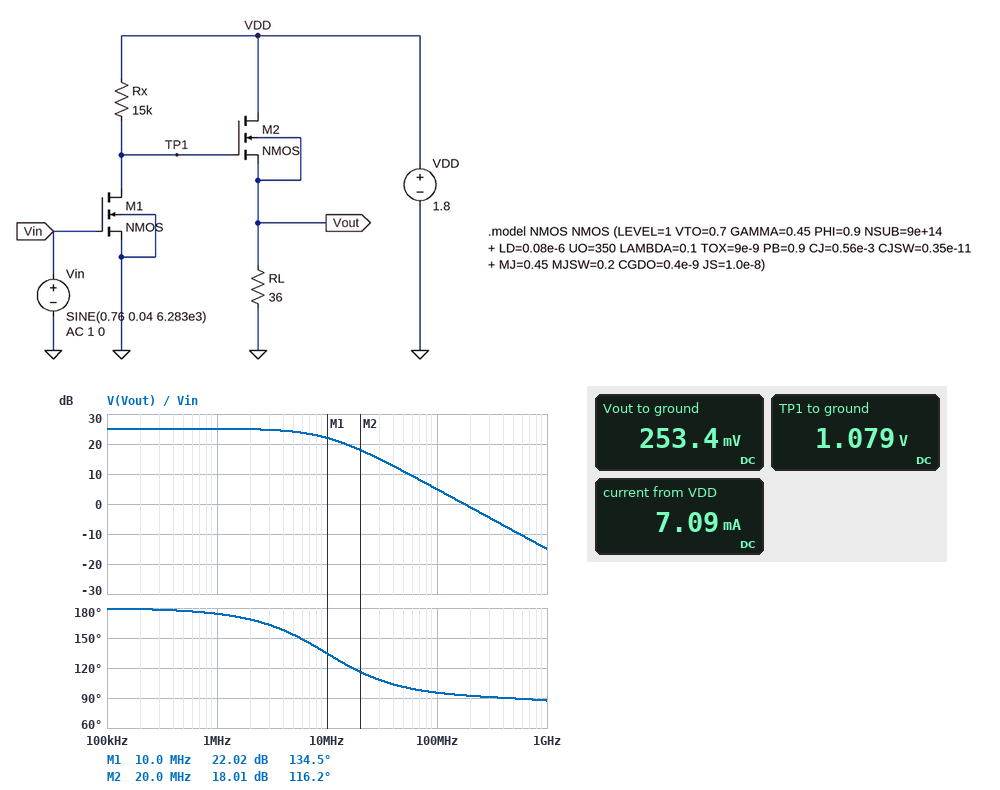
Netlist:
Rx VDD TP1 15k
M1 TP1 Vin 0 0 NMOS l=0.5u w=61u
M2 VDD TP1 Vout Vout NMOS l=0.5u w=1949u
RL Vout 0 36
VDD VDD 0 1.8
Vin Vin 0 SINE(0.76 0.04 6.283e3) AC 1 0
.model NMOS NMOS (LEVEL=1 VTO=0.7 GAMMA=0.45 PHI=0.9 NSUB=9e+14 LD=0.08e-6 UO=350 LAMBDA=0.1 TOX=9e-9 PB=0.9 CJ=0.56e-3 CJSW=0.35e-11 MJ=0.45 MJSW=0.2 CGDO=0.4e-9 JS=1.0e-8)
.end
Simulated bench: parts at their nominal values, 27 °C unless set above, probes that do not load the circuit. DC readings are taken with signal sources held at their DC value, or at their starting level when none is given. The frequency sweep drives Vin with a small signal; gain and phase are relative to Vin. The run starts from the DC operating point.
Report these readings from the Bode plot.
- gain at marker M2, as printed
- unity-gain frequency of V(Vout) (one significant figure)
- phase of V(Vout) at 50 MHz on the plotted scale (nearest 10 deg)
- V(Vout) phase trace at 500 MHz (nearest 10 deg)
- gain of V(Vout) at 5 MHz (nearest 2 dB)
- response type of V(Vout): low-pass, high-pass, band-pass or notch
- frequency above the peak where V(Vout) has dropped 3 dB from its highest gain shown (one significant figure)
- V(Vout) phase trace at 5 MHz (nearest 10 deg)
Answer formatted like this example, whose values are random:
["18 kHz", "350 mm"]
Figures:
["18.01 dB", "200 MHz", "100 deg", "90 deg", "24 dB", "low-pass", "10 MHz", "150 deg"]
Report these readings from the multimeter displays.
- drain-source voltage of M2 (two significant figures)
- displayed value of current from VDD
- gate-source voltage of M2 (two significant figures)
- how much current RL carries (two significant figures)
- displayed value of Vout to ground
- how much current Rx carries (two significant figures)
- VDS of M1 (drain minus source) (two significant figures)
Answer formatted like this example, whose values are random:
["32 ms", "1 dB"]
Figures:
["1.5 V", "7.09 mA", "830 mV", "7.0 mA", "253.4 mV", "48 µA", "1.1 V"]
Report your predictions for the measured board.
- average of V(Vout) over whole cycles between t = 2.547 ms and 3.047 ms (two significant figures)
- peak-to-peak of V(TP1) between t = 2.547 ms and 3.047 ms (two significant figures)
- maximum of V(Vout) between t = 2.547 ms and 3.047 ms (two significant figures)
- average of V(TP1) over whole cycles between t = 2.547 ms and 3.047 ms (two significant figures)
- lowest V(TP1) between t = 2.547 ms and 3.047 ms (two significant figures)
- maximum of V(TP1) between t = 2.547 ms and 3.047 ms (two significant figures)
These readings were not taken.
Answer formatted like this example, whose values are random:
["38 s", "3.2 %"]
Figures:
["330 mV", "1.6 V", "790 mV", "970 mV", "77 mV", "1.7 V"]
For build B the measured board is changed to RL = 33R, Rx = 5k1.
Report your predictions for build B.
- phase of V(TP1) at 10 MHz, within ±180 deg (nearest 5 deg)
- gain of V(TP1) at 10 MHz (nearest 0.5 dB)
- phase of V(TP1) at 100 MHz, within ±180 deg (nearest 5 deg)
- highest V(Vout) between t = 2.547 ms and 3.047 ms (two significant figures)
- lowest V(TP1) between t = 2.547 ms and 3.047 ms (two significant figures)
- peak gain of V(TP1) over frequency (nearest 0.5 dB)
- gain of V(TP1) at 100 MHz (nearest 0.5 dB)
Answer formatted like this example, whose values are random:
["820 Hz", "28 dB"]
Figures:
["160 deg", "18.0 dB", "105 deg", "830 mV", "1.1 V", "18.5 dB", "7.5 dB"]
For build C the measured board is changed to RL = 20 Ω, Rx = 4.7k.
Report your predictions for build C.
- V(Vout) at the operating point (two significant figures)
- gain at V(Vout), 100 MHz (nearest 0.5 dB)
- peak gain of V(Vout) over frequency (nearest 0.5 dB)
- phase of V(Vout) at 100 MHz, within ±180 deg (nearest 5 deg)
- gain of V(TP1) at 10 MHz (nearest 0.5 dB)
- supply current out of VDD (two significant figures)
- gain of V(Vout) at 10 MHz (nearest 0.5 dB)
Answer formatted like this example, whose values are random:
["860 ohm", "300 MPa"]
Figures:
["600 mV", "5.5 dB", "16.0 dB", "105 deg", "17.5 dB", "30 mA", "15.5 dB"]
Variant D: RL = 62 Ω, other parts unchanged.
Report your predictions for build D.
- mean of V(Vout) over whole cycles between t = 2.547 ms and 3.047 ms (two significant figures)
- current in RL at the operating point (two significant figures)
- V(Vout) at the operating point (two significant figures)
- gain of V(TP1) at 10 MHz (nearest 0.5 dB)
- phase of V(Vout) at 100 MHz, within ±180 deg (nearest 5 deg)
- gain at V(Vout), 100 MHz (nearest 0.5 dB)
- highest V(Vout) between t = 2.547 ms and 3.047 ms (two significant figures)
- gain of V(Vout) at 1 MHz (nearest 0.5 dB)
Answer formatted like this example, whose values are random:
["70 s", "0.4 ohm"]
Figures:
["350 mV", "4.5 mA", "280 mV", "24.5 dB", "95 deg", "6.0 dB", "840 mV", "25.5 dB"]
